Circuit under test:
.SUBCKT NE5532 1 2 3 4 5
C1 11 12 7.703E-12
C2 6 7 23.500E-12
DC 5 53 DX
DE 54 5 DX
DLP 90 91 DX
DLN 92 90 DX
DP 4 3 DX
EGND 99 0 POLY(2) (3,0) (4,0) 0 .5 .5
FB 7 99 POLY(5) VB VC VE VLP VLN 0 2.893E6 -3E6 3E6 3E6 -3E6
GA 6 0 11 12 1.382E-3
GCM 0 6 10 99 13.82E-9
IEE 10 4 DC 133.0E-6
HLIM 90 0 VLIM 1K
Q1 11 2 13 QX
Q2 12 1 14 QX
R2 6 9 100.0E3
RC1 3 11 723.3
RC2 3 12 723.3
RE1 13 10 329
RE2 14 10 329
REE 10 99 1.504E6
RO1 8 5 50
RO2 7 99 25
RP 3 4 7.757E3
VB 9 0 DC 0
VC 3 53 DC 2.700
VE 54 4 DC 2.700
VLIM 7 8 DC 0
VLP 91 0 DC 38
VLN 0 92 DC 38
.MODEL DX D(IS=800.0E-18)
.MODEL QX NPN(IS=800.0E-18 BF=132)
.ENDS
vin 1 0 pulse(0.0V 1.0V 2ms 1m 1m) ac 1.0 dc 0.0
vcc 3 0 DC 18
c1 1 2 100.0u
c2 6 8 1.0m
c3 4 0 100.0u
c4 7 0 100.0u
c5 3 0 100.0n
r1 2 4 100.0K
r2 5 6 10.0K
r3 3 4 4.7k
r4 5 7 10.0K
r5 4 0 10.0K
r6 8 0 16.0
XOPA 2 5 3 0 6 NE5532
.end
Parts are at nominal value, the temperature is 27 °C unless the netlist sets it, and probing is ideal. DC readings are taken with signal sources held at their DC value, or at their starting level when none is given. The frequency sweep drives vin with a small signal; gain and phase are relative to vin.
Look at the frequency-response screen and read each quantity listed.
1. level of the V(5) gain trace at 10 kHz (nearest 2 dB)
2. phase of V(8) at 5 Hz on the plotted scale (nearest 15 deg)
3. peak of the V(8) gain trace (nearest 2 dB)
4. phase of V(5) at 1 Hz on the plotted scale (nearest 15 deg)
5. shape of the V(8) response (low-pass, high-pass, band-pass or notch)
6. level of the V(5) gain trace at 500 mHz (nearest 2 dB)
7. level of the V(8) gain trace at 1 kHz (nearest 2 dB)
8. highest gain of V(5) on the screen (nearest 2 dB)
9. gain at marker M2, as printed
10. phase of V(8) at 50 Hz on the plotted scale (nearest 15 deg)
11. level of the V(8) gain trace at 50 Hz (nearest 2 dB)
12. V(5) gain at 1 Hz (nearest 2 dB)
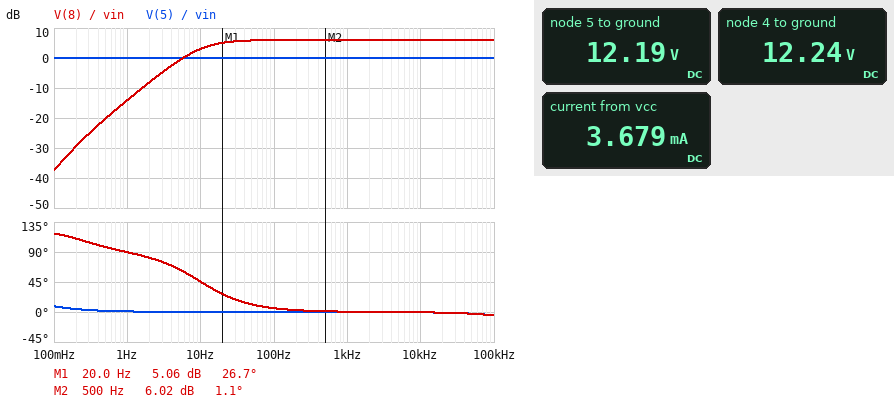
0 dB
60 deg
6 dB
0 deg
high-pass
0 dB
6 dB
0 dB
6.02 dB
15 deg
6 dB
0 dB
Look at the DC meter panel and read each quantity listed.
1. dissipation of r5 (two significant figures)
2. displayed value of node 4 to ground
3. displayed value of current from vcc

15 mW
12.24 V
3.679 mA
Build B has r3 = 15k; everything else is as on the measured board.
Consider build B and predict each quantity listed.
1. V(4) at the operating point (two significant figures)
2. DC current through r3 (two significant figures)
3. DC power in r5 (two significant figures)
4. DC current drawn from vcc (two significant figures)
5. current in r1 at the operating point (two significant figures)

7.2 V
720 µA
5.2 mW
3.2 mA
490 nA
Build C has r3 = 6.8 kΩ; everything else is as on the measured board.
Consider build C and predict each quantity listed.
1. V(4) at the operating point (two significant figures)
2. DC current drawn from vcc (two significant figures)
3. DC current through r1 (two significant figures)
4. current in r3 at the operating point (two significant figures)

11 V
3.5 mA
500 nA
1.1 mA
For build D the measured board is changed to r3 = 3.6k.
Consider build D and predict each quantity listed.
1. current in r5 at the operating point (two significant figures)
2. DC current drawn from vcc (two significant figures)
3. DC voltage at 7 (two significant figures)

1.3 mA
3.8 mA
13 V
